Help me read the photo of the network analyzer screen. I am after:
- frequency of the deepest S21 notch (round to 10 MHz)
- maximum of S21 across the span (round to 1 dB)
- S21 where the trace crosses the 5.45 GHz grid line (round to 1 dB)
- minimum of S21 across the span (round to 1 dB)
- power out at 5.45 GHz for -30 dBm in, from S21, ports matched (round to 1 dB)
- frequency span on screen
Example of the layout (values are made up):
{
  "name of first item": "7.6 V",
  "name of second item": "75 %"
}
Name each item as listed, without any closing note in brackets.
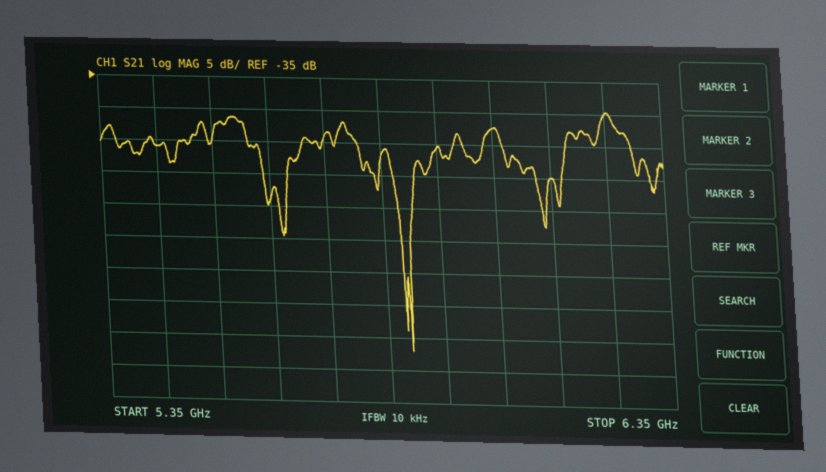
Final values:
{
  "frequency of the deepest S21 notch": "5.89 GHz",
  "maximum of S21 across the span": "-40 dB",
  "S21 where the trace crosses the 5.45 GHz grid line": "-46 dB",
  "minimum of S21 across the span": "-77 dB",
  "power out at 5.45 GHz for -30 dBm in, from S21, ports matched": "-76 dBm",
  "frequency span on screen": "1 GHz"
}
